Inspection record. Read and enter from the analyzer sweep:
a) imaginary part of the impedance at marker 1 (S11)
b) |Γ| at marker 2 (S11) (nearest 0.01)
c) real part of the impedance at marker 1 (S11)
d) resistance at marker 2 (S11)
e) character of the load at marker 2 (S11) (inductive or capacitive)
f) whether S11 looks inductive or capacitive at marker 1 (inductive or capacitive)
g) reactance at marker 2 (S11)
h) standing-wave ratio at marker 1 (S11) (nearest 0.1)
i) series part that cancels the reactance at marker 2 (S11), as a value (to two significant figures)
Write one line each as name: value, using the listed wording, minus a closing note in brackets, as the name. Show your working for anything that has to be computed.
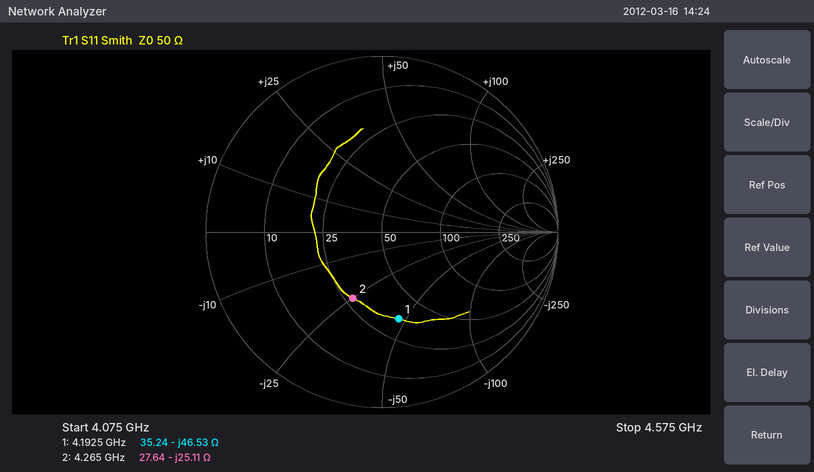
imaginary part of the impedance at marker 1: -46.53 Ω
|Γ| at marker 2 (S11): 0.41
real part of the impedance at marker 1: 35.24 Ω
resistance at marker 2: 27.64 Ω
character of the load at marker 2 (S11): capacitive
whether S11 looks inductive or capacitive at marker 1: capacitive
reactance at marker 2: -25.11 Ω
standing-wave ratio at marker 1 (S11): 3.0
series part that cancels the reactance at marker 2 (S11), as a value: L = 25.11 Ω/(2π × 4.265 GHz) ≈ 937 pH, so 940 pH to two significant figures
